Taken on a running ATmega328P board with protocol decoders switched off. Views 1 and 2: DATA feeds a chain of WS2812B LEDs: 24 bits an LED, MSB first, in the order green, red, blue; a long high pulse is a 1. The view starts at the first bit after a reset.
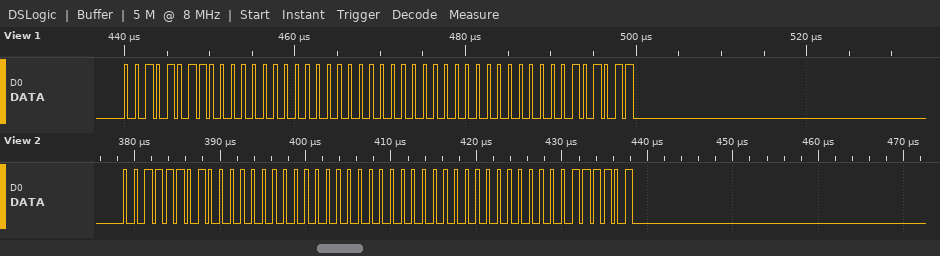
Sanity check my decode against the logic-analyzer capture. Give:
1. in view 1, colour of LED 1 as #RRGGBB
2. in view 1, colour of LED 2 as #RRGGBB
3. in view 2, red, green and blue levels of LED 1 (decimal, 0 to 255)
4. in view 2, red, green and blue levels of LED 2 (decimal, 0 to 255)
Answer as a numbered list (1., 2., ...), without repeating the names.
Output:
1. #002B00
2. #00002B
3. 0, 61, 0
4. 0, 0, 61
